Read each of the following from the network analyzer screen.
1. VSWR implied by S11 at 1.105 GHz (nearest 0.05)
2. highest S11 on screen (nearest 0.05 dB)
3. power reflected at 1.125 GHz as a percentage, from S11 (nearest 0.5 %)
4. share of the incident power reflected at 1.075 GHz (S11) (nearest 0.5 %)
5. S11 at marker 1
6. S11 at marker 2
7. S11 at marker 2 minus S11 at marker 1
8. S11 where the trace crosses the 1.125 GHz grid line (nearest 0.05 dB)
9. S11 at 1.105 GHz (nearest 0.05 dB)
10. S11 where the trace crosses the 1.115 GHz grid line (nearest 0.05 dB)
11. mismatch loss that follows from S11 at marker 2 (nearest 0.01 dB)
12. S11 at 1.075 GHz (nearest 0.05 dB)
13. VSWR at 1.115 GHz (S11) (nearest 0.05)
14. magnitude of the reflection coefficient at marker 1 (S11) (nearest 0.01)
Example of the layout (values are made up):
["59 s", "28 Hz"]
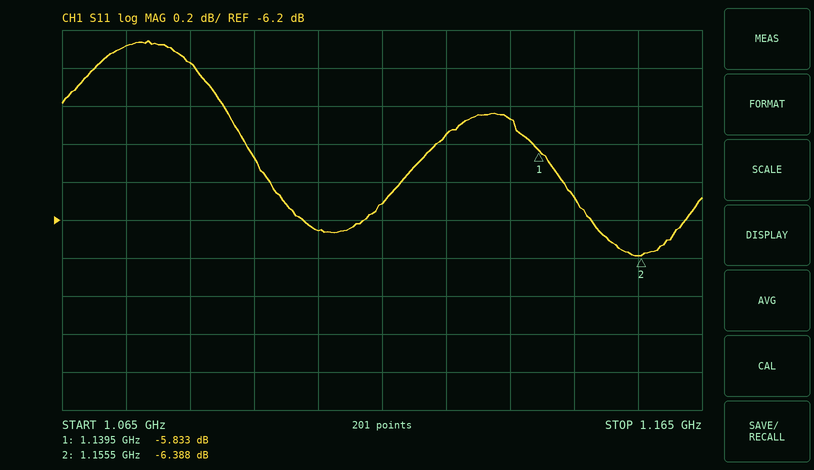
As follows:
["2.90", "-5.25 dB", "26.5 %", "29.5 %", "-5.833 dB", "-6.388 dB", "-0.555 dB", "-5.75 dB", "-6.25 dB", "-6.10 dB", "1.13 dB", "-5.30 dB", "2.95", "0.51"]
